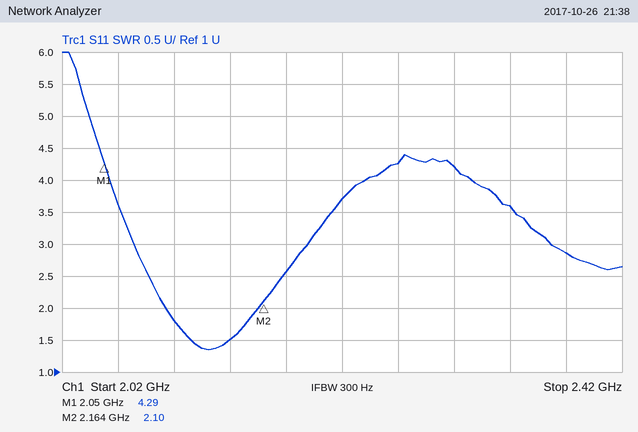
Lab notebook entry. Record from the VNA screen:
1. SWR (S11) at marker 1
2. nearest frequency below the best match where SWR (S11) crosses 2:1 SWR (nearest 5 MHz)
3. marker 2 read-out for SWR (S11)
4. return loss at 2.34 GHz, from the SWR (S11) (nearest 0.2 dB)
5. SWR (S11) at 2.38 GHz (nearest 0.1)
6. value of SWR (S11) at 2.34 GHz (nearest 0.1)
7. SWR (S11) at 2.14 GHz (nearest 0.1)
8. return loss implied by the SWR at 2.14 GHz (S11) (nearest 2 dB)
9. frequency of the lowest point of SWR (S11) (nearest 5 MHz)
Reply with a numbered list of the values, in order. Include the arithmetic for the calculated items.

1. 4.29
2. 2.095 GHz
3. 2.10
4. −20 log10((3.6 − 1)/(3.6 + 1)) ≈ 5.0 dB
5. 2.9
6. 3.6
7. 1.5
8. −20 log10((1.5 − 1)/(1.5 + 1)) ≈ 14 dB
9. 2.125 GHz
